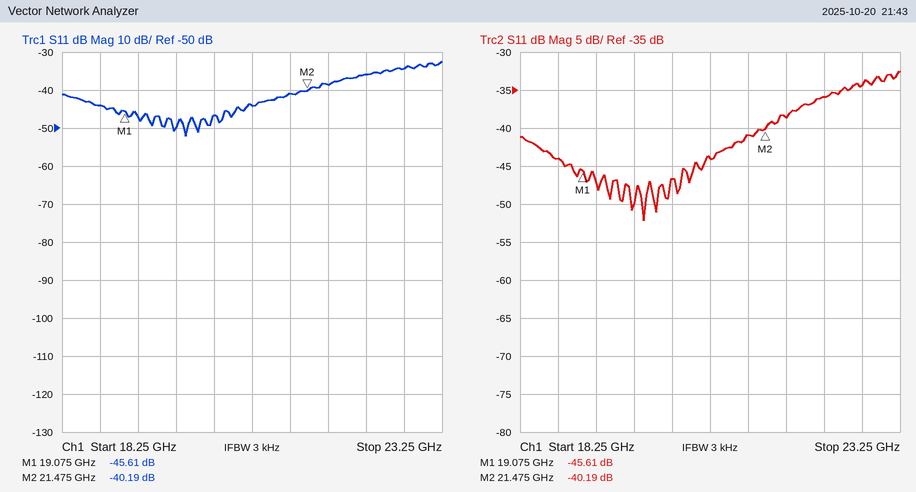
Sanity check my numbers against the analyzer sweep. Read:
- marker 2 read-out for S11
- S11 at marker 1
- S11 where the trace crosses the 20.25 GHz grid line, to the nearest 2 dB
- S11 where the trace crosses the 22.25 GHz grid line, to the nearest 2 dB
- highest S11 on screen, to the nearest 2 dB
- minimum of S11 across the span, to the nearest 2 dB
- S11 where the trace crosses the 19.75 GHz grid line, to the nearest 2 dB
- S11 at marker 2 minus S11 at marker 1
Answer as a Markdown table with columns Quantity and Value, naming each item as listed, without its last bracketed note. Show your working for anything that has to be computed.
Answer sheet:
| Quantity | Value |
|---|---|
| marker 2 read-out for S11 | -40.19 dB |
| S11 at marker 1 | -45.61 dB |
| S11 where the trace crosses the 20.25 GHz grid line, to the nearest 2 dB | -46 dB |
| S11 where the trace crosses the 22.25 GHz grid line, to the nearest 2 dB | -36 dB |
| highest S11 on screen, to the nearest 2 dB | -32 dB |
| minimum of S11 across the span, to the nearest 2 dB | -52 dB |
| S11 where the trace crosses the 19.75 GHz grid line, to the nearest 2 dB | -50 dB |
| S11 at marker 2 minus S11 at marker 1 | -40.19 − (-45.61) = 5.42 dB |
